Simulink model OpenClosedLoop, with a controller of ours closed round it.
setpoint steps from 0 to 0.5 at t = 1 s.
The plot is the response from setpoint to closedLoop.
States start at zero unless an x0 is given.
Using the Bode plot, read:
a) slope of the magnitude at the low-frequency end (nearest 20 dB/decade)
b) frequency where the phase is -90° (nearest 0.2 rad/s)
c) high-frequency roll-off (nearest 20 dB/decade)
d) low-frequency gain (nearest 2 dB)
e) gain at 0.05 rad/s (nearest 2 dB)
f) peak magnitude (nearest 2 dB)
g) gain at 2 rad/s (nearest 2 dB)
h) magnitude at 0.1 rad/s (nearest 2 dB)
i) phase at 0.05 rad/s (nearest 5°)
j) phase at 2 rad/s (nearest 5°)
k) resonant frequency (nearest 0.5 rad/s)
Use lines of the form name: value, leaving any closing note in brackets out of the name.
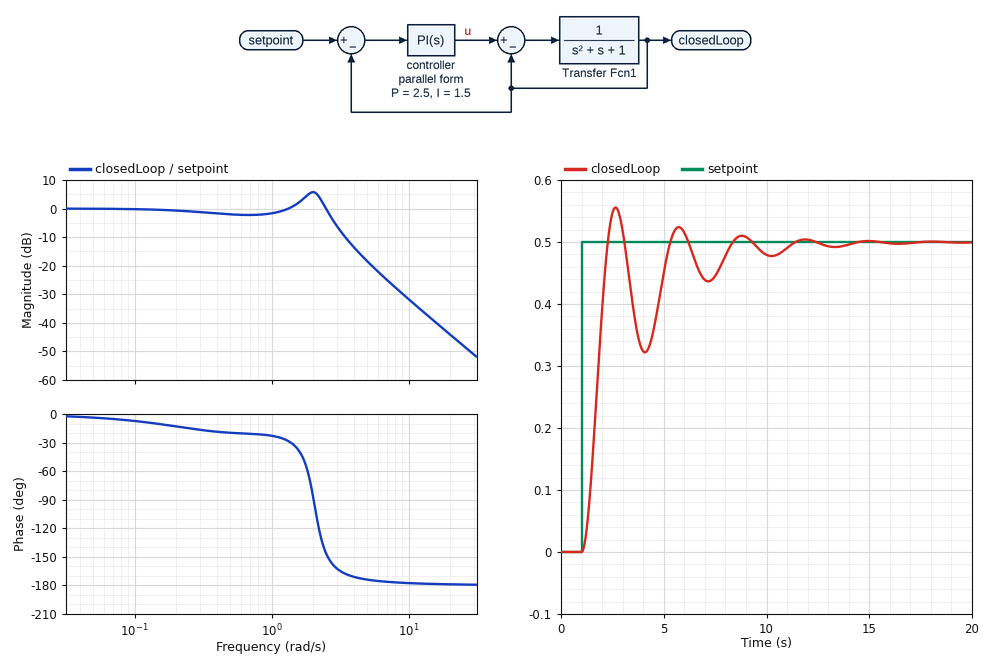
slope of the magnitude at the low-frequency end: 0 dB/decade
frequency where the phase is -90°: 2.0 rad/s
high-frequency roll-off: -40 dB/decade
low-frequency gain: 0 dB
gain at 0.05 rad/s: 0 dB
peak magnitude: 6 dB
gain at 2 rad/s: 6 dB
magnitude at 0.1 rad/s: 0 dB
phase at 0.05 rad/s: -5°
phase at 2 rad/s: -85°
resonant frequency: 2.0 rad/s
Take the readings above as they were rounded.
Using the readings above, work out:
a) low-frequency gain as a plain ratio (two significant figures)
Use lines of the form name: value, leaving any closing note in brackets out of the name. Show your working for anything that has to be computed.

low-frequency gain as a plain ratio: 10^(0 / 20) = 1.0
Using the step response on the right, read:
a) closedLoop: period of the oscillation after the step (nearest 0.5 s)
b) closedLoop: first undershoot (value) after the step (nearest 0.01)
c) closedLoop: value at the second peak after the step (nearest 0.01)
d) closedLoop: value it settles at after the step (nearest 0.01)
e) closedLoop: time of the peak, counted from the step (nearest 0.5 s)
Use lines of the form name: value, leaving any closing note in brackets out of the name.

closedLoop: period of the oscillation after the step: 3.0 s
closedLoop: first undershoot (value) after the step: 0.32
closedLoop: value at the second peak after the step: 0.52
closedLoop: value it settles at after the step: 0.50
closedLoop: time of the peak, counted from the step: 1.5 s
